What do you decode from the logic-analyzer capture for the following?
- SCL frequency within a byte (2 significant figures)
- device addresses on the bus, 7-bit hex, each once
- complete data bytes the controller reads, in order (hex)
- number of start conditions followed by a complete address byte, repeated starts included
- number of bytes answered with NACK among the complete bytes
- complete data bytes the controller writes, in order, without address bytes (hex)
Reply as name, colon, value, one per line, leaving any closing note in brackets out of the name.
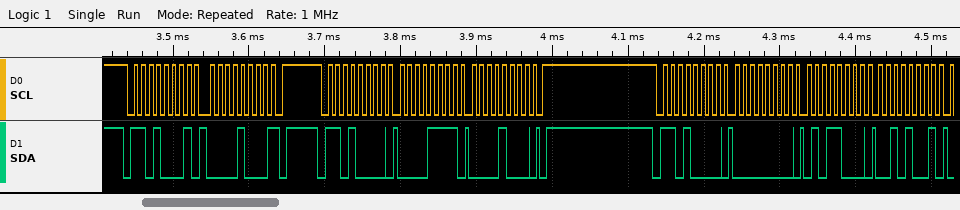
SCL frequency within a byte: 100 kHz
device addresses on the bus, 7-bit hex, each once: 0x68
complete data bytes the controller reads, in order: 08
number of start conditions followed by a complete address byte, repeated starts included: 3
number of bytes answered with NACK among the complete bytes: 1
complete data bytes the controller writes, in order, without address bytes: 0F 08 00 58 29
